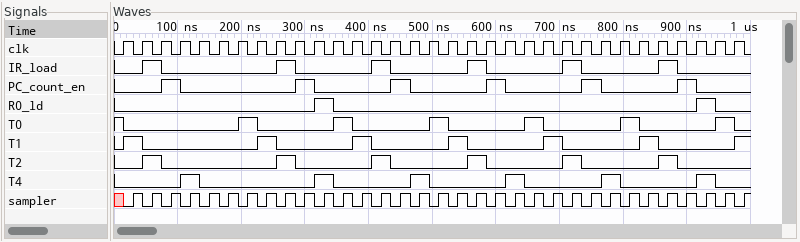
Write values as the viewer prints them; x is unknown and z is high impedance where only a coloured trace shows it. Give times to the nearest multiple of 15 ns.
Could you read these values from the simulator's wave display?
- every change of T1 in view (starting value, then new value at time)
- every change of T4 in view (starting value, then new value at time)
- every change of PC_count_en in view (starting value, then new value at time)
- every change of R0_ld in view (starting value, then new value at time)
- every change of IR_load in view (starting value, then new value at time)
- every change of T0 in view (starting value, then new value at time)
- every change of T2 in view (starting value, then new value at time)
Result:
0, 1 at 15 ns, 0 at 45 ns, 1 at 225 ns, 0 at 255 ns, 1 at 375 ns, 0 at 405 ns, 1 at 525 ns, 0 at 555 ns, 1 at 675 ns, 0 at 705 ns, 1 at 825 ns, 0 at 855 ns, 1 at 975 ns
0, 1 at 105 ns, 0 at 135 ns, 1 at 315 ns, 0 at 345 ns, 1 at 465 ns, 0 at 495 ns, 1 at 615 ns, 0 at 645 ns, 1 at 765 ns, 0 at 795 ns, 1 at 915 ns, 0 at 945 ns
0, 1 at 75 ns, 0 at 105 ns, 1 at 285 ns, 0 at 315 ns, 1 at 435 ns, 0 at 465 ns, 1 at 585 ns, 0 at 615 ns, 1 at 735 ns, 0 at 765 ns, 1 at 885 ns, 0 at 915 ns
0, 1 at 315 ns, 0 at 345 ns, 1 at 915 ns, 0 at 945 ns
0, 1 at 45 ns, 0 at 75 ns, 1 at 255 ns, 0 at 285 ns, 1 at 405 ns, 0 at 435 ns, 1 at 555 ns, 0 at 585 ns, 1 at 705 ns, 0 at 735 ns, 1 at 855 ns, 0 at 885 ns
1, 0 at 15 ns, 1 at 195 ns, 0 at 225 ns, 1 at 345 ns, 0 at 375 ns, 1 at 495 ns, 0 at 525 ns, 1 at 645 ns, 0 at 675 ns, 1 at 795 ns, 0 at 825 ns, 1 at 945 ns, 0 at 975 ns
0, 1 at 45 ns, 0 at 75 ns, 1 at 255 ns, 0 at 285 ns, 1 at 405 ns, 0 at 435 ns, 1 at 555 ns, 0 at 585 ns, 1 at 705 ns, 0 at 735 ns, 1 at 855 ns, 0 at 885 ns
